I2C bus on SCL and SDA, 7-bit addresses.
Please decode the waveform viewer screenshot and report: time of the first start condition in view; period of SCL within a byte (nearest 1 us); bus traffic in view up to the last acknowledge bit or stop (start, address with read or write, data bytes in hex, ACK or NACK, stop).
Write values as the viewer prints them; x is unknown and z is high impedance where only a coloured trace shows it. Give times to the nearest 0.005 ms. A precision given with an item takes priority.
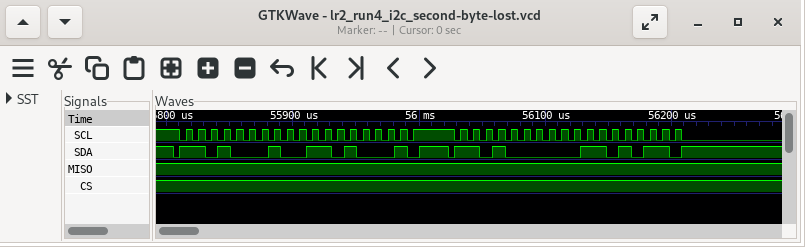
55.805 ms
10 us
start, address 68 read ACK, 68 NACK, stop, start, address 68 write ACK, 6B ACK
